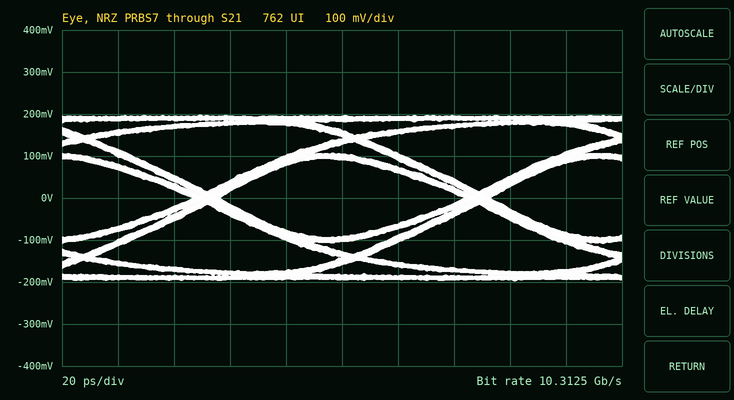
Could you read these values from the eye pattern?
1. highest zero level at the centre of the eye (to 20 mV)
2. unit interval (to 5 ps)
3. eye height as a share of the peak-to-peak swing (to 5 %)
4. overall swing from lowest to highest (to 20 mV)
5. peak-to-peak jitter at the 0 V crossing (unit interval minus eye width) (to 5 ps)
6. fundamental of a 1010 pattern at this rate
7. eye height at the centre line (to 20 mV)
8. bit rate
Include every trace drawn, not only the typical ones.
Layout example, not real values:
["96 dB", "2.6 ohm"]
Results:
["-100 mV", "95 ps", "45 %", "400 mV", "10 ps", "5.15625 GHz", "180 mV", "10.3125 Gb/s"]
